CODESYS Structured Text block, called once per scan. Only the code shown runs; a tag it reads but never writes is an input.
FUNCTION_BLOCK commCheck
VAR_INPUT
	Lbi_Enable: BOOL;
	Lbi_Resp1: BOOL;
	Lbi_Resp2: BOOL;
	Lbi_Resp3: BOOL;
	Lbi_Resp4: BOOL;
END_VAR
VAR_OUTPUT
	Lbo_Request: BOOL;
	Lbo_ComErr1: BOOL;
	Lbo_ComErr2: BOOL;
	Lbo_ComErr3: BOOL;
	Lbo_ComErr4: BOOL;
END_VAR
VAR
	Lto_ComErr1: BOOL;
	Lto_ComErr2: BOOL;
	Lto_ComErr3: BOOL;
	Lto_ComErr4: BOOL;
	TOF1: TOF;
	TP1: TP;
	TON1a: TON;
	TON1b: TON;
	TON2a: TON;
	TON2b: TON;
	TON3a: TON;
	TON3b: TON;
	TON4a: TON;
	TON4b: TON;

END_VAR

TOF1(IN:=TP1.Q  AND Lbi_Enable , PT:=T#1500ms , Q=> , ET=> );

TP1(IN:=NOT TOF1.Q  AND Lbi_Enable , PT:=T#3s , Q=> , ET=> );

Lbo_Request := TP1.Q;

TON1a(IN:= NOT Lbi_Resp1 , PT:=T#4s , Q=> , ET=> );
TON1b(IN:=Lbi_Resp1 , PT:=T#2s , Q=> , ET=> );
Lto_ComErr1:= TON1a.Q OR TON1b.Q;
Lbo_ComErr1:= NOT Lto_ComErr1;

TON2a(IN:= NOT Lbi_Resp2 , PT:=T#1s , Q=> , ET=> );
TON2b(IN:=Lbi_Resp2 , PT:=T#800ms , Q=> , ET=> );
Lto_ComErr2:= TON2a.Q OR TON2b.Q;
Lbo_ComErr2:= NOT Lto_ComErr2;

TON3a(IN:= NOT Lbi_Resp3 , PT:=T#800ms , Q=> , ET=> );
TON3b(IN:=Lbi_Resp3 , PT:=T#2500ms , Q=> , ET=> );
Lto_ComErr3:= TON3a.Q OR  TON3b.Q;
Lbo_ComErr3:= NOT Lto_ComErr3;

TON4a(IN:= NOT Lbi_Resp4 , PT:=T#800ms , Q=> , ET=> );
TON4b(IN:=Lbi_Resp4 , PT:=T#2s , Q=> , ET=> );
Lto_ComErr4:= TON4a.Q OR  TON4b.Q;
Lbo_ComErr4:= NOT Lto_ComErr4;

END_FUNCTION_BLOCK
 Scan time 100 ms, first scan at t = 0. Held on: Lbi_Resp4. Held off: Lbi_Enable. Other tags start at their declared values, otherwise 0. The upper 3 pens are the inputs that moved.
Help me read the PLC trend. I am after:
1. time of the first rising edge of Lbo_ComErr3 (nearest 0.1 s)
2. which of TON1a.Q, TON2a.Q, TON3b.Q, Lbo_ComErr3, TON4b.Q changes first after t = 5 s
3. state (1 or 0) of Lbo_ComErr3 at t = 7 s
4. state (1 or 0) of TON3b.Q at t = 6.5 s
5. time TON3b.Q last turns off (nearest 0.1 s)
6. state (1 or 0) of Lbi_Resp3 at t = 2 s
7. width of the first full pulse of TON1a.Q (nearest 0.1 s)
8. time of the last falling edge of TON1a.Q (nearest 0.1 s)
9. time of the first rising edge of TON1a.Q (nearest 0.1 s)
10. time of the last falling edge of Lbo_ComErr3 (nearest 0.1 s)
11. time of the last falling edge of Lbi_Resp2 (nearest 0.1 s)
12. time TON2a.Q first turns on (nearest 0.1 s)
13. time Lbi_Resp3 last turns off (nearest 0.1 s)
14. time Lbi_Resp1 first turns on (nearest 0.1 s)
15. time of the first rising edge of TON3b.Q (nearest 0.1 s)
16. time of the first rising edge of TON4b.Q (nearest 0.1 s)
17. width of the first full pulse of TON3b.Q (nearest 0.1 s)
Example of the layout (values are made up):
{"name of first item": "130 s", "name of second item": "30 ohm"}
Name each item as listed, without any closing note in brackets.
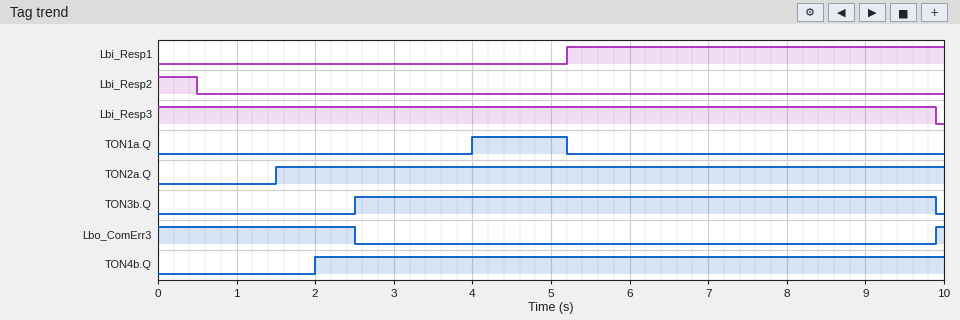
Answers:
{"time of the first rising edge of Lbo_ComErr3": "9.9 s", "which of TON1a.Q, TON2a.Q, TON3b.Q, Lbo_ComErr3, TON4b.Q changes first after t = 5 s": "TON1a.Q", "state (1 or 0) of Lbo_ComErr3 at t = 7 s": "0", "state (1 or 0) of TON3b.Q at t = 6.5 s": "1", "time TON3b.Q last turns off": "9.9 s", "state (1 or 0) of Lbi_Resp3 at t = 2 s": "1", "width of the first full pulse of TON1a.Q": "1.2 s", "time of the last falling edge of TON1a.Q": "5.2 s", "time of the first rising edge of TON1a.Q": "4.0 s", "time of the last falling edge of Lbo_ComErr3": "2.5 s", "time of the last falling edge of Lbi_Resp2": "0.5 s", "time TON2a.Q first turns on": "1.5 s", "time Lbi_Resp3 last turns off": "9.9 s", "time Lbi_Resp1 first turns on": "5.2 s", "time of the first rising edge of TON3b.Q": "2.5 s", "time of the first rising edge of TON4b.Q": "2.0 s", "width of the first full pulse of TON3b.Q": "7.4 s"}
